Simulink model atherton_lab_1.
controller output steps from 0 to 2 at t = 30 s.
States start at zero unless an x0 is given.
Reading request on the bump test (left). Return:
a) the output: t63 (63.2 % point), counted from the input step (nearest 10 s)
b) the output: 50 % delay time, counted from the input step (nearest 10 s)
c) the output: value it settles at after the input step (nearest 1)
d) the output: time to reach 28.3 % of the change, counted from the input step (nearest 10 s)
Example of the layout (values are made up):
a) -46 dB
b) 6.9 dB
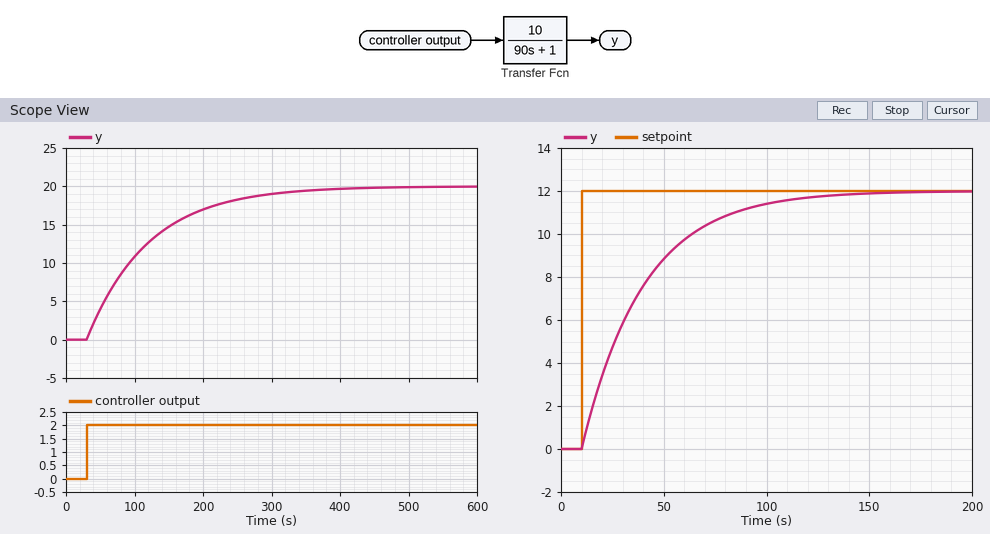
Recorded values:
a) 90 s
b) 60 s
c) 20
d) 30 s
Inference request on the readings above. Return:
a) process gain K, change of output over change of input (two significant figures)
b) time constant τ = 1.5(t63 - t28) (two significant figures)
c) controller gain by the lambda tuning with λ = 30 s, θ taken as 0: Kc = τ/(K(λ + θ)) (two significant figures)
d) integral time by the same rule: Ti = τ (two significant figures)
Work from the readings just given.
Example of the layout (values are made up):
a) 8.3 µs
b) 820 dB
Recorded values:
a) 10
b) 90 s
c) 0.30
d) 90 s
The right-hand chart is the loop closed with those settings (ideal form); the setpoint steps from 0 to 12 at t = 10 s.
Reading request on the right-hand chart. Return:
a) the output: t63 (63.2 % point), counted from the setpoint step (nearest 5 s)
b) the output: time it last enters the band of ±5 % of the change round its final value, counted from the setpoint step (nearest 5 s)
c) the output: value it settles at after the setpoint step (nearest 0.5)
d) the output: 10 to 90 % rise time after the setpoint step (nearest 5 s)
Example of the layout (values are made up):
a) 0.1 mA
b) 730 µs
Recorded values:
a) 30 s
b) 90 s
c) 12.0
d) 65 s
